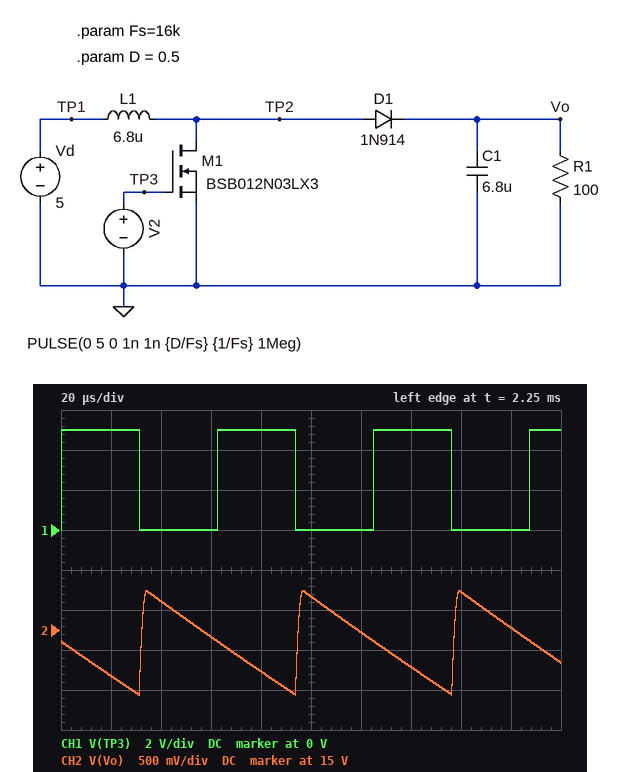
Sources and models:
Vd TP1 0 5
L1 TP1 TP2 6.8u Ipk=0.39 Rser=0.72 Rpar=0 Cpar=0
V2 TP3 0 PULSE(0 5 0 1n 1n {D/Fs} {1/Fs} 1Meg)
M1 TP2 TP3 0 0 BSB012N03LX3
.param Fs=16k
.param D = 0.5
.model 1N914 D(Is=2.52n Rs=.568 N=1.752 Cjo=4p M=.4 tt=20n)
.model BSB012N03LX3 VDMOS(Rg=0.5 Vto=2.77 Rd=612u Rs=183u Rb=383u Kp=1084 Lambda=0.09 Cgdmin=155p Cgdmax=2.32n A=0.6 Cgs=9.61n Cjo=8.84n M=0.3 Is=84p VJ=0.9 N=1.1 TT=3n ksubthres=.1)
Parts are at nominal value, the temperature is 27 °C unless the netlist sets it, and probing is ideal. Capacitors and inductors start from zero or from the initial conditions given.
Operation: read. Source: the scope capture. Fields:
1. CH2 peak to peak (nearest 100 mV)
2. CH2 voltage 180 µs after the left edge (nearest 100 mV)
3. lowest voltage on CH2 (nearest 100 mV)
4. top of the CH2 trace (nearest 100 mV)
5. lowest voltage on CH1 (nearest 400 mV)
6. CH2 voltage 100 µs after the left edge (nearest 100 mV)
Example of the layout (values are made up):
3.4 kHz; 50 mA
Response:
1.3 V; 15.0 V; 14.2 V; 15.5 V; 0 V; 15.4 V
